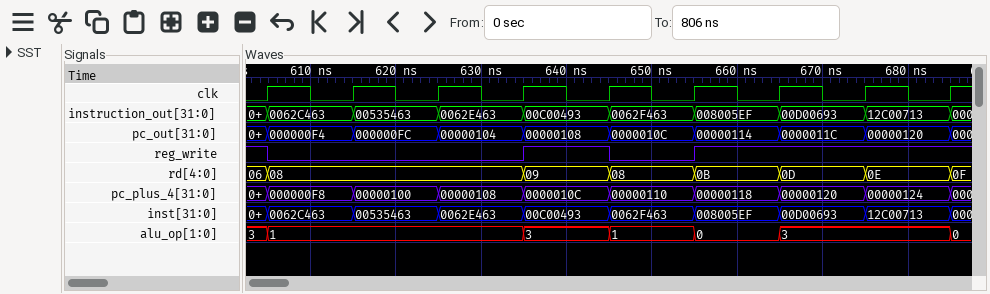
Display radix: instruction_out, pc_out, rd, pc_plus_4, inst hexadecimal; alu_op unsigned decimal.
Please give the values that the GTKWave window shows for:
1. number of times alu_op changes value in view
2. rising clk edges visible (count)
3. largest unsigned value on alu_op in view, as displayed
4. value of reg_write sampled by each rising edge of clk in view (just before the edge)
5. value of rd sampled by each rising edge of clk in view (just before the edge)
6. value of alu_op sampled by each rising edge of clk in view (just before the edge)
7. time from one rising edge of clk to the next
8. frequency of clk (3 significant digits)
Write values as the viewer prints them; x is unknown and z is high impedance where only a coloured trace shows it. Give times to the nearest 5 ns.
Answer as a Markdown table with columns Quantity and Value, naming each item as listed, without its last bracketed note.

| Quantity | Value |
|---|---|
| number of times alu_op changes value in view | 6 |
| rising clk edges visible | 9 |
| largest unsigned value on alu_op in view, as displayed | 3 |
| value of reg_write sampled by each rising edge of clk in view | 1 0 0 0 1 0 1 1 1 |
| value of rd sampled by each rising edge of clk in view | 06, 08, 08, 08, 09, 08, 0B, 0D, 0E |
| value of alu_op sampled by each rising edge of clk in view | 3, 1, 1, 1, 3, 1, 0, 3, 3 |
| time from one rising edge of clk to the next | 10 ns |
| frequency of clk | 100 MHz |
